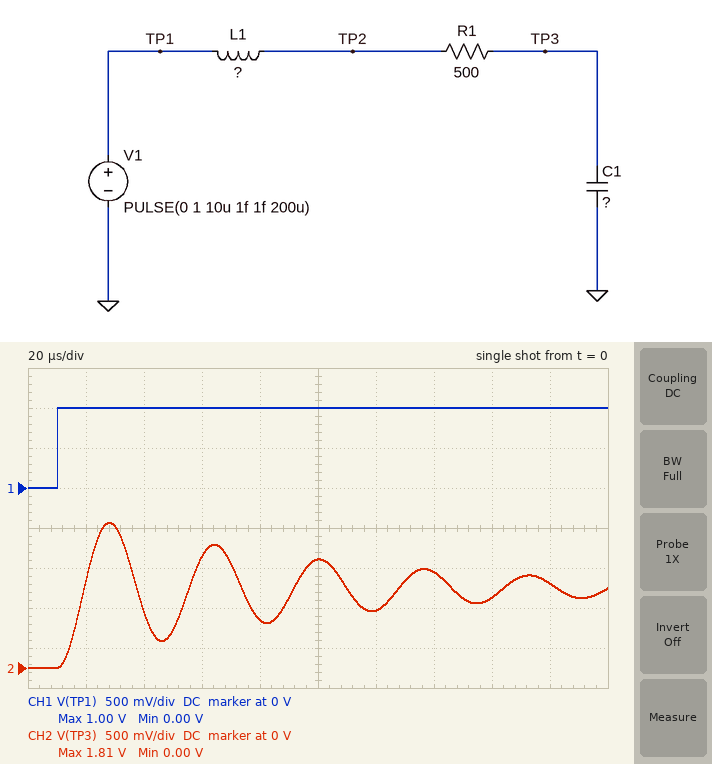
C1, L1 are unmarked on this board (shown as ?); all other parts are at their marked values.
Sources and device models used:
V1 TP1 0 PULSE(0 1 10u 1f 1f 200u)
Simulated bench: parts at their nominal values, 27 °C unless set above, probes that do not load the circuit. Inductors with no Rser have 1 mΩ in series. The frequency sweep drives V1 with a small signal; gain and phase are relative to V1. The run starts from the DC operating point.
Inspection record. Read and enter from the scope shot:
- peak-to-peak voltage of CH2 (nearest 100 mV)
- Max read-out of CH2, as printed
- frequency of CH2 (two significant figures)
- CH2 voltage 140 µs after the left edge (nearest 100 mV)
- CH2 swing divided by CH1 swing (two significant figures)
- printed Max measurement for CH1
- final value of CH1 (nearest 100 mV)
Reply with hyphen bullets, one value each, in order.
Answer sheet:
- 1.8 V
- 1.81 V
- 28 kHz
- 1.2 V
- 1.8
- 1.00 V
- 1.0 V
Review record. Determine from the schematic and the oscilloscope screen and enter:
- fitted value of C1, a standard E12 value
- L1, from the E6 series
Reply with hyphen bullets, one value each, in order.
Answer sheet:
- 1.5 nF
- 22 mH
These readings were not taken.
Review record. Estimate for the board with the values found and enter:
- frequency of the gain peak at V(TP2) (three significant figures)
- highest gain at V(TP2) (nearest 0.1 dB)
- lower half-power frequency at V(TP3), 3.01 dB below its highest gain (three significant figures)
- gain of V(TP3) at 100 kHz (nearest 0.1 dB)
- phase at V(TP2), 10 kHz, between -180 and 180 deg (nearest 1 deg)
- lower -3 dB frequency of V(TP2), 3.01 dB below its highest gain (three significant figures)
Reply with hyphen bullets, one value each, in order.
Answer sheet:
- 27.6 kHz
- 17.8 dB
- 25.7 kHz
- -21.6 dB
- 0 deg
- 25.7 kHz
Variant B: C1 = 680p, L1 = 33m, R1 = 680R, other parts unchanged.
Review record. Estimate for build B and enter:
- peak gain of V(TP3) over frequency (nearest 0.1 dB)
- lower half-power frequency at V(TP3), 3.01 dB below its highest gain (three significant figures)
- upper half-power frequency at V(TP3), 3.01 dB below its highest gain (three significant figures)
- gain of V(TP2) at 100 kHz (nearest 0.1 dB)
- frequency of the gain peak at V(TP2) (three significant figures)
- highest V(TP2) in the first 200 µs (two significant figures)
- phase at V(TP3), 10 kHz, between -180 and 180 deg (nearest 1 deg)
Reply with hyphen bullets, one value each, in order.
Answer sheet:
- 20.2 dB
- 31.8 kHz
- 35.1 kHz
- -17.6 dB
- 33.5 kHz
- 1.9 V
- -2 deg
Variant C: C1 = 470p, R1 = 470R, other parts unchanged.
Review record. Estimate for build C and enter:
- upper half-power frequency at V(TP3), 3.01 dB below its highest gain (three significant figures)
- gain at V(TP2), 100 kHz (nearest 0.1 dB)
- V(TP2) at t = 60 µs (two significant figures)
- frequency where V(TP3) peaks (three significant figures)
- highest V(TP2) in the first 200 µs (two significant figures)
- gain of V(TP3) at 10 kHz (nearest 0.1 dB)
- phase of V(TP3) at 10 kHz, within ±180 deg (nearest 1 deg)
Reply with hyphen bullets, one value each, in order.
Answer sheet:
- 51.1 kHz
- -9.7 dB
- 1.6 V
- 49.4 kHz
- 1.9 V
- 0.4 dB
- -1 deg
